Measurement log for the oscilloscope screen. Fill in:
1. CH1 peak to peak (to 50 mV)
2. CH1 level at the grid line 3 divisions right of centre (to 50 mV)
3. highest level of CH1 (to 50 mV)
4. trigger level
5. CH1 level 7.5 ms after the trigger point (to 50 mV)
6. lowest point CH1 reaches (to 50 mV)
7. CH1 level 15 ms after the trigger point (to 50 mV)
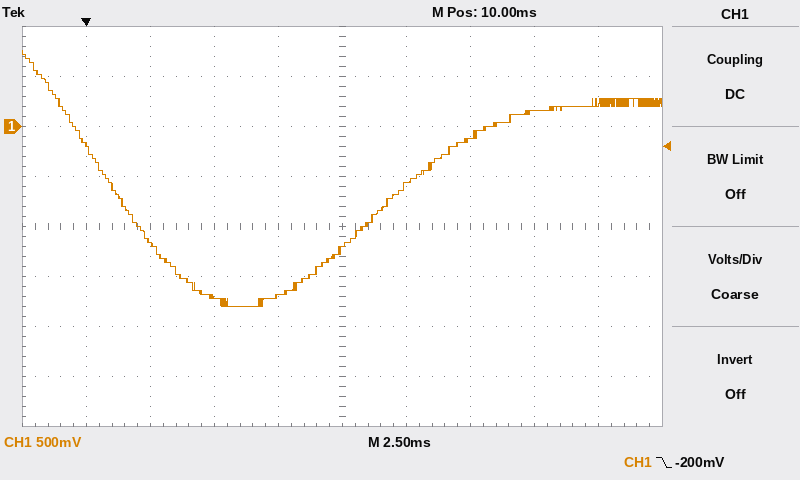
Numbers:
2.55 V
150 mV
750 mV
-200 mV
-1.70 V
-1.80 V
-150 mV
